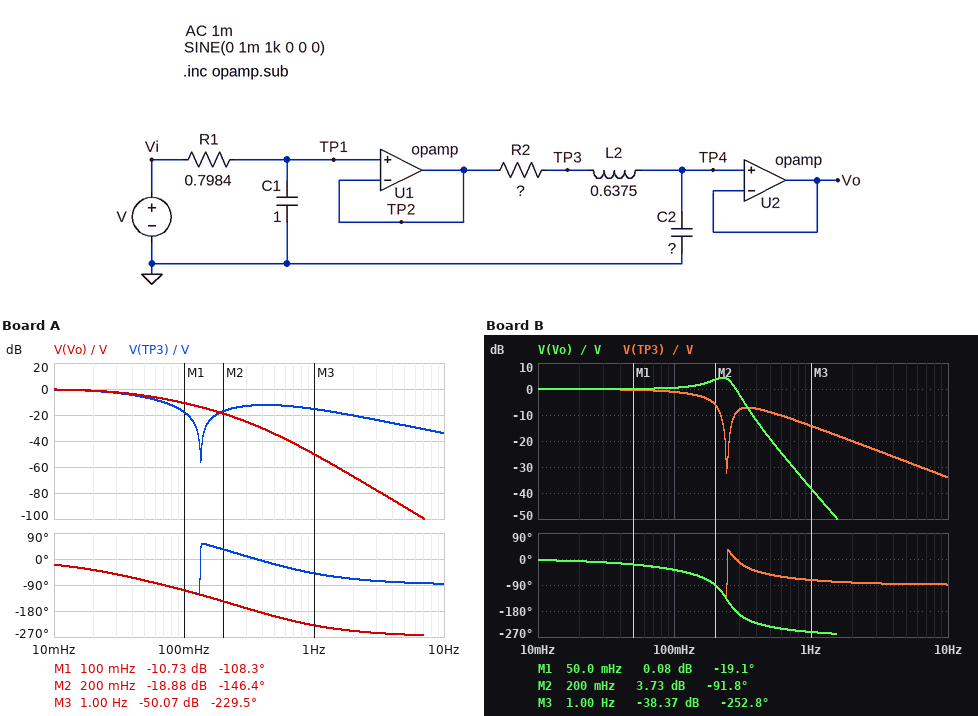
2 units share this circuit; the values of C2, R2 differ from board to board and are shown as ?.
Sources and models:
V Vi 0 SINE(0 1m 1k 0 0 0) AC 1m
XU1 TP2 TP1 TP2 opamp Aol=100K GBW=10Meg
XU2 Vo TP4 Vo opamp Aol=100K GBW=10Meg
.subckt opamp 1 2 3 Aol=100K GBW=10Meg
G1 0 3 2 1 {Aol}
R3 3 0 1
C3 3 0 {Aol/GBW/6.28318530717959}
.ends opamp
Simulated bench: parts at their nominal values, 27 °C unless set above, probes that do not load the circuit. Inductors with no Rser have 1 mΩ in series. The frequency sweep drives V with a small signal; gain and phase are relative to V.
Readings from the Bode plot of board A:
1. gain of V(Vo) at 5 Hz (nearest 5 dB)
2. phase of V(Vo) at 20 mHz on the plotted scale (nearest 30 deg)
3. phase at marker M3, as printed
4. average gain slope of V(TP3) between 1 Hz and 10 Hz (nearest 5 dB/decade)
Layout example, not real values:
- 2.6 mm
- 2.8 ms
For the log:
- -90 dB
- -30 deg
- -229.5 deg
- -20 dB/decade
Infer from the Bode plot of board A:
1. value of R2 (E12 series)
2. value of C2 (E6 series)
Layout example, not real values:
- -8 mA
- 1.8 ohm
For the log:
- 2.2 Ω
- 2.2 F
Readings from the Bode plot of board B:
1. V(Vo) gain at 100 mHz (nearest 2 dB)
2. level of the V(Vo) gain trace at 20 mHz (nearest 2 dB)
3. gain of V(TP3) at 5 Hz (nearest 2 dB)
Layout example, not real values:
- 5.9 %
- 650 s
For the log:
- 0 dB
- 0 dB
- -28 dB
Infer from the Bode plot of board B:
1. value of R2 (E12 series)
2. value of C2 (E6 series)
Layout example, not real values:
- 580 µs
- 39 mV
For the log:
- 0.39 Ω
- 680 mF
